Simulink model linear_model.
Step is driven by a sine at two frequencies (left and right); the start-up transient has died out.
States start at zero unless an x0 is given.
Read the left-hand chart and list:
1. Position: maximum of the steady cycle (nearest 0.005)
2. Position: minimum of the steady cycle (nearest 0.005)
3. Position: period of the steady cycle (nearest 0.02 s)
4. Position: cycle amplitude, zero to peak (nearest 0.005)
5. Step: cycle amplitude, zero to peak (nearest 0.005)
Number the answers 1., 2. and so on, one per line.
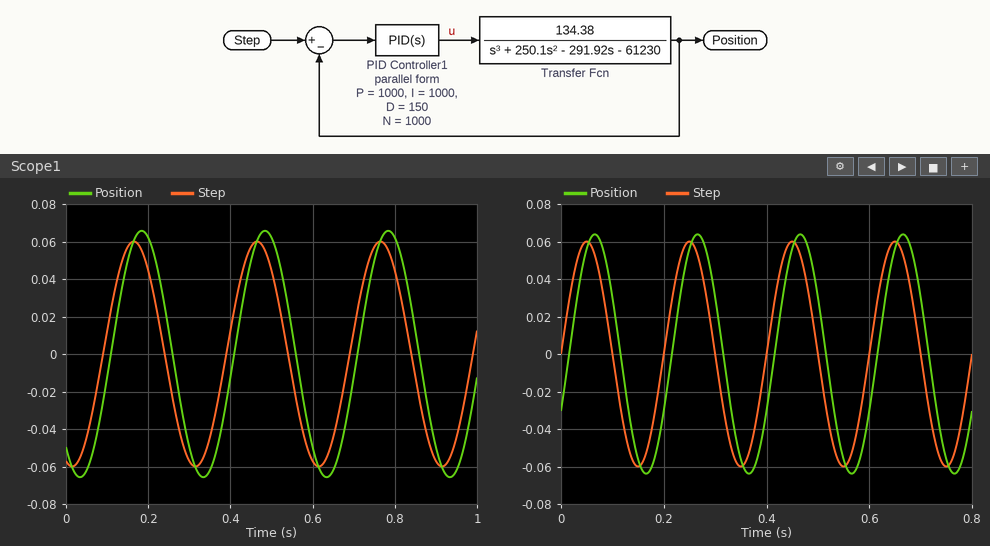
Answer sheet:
1. 0.065
2. -0.065
3. 0.30 s
4. 0.065
5. 0.060
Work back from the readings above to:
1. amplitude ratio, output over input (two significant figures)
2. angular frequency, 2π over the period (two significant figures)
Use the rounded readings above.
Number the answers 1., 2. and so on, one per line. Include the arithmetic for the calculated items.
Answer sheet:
1. 0.065 / 0.06 = 1.1
2. 2π / 0.3 = 21 rad/s
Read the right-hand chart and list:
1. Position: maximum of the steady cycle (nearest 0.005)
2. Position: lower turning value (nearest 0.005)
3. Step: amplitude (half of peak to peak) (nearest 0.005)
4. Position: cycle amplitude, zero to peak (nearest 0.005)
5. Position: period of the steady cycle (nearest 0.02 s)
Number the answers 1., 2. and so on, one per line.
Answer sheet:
1. 0.065
2. -0.065
3. 0.060
4. 0.065
5. 0.20 s
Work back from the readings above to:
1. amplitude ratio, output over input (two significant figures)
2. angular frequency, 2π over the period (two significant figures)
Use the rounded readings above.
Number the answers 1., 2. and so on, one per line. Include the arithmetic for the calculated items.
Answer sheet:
1. 0.065 / 0.06 = 1.1
2. 2π / 0.2 = 31 rad/s
